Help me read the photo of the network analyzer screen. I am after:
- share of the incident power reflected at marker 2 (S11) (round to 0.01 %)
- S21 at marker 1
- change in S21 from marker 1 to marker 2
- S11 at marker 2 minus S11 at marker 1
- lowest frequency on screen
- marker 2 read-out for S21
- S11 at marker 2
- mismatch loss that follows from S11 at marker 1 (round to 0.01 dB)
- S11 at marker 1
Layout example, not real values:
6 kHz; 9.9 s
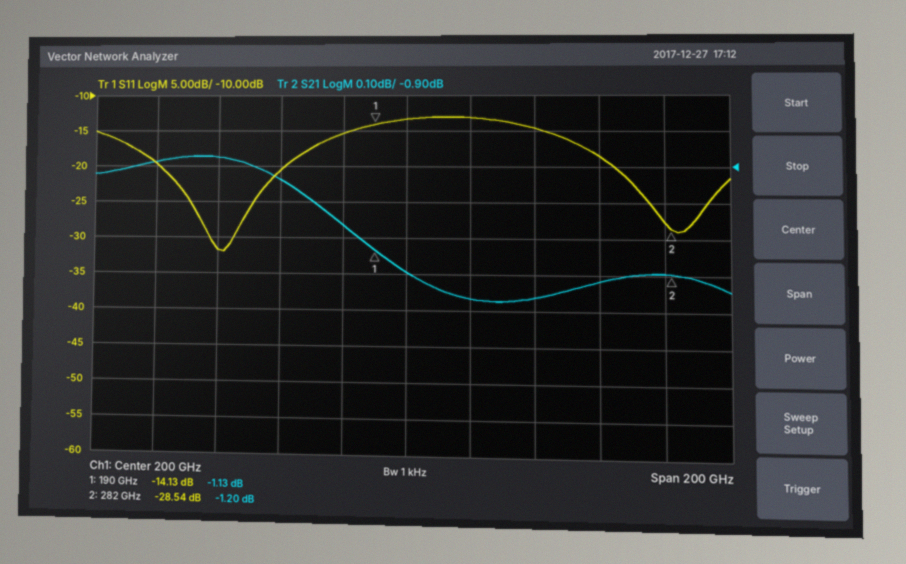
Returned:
0.14 %; -1.13 dB; -0.07 dB; -14.41 dB; 100 GHz; -1.20 dB; -28.54 dB; 0.17 dB; -14.13 dB
